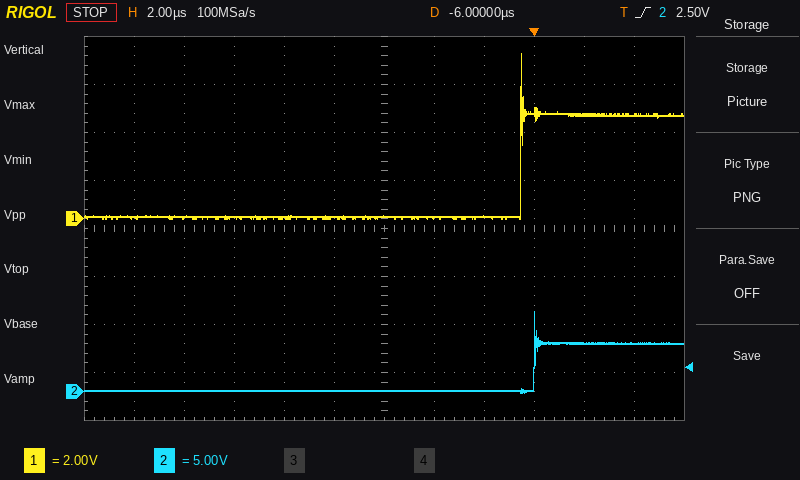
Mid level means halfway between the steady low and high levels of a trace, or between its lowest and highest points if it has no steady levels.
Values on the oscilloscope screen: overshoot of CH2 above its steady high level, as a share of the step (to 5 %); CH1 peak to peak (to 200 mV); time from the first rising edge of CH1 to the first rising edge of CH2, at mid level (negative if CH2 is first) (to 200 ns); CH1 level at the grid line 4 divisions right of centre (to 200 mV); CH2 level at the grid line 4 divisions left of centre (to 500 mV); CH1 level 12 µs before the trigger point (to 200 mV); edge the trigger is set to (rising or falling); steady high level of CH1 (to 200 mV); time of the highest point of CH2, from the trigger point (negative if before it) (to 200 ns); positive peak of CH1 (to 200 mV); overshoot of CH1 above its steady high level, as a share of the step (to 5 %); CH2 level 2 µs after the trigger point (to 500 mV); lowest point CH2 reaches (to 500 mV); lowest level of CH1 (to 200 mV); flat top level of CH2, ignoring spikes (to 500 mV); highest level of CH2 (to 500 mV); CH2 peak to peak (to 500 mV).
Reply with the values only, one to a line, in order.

65 %
6.8 V
+600 ns
4.4 V
0.0 V
0.0 V
rising
4.4 V
0.0 µs
6.8 V
60 %
5.0 V
0.0 V
0.0 V
5.0 V
8.5 V
8.5 V
